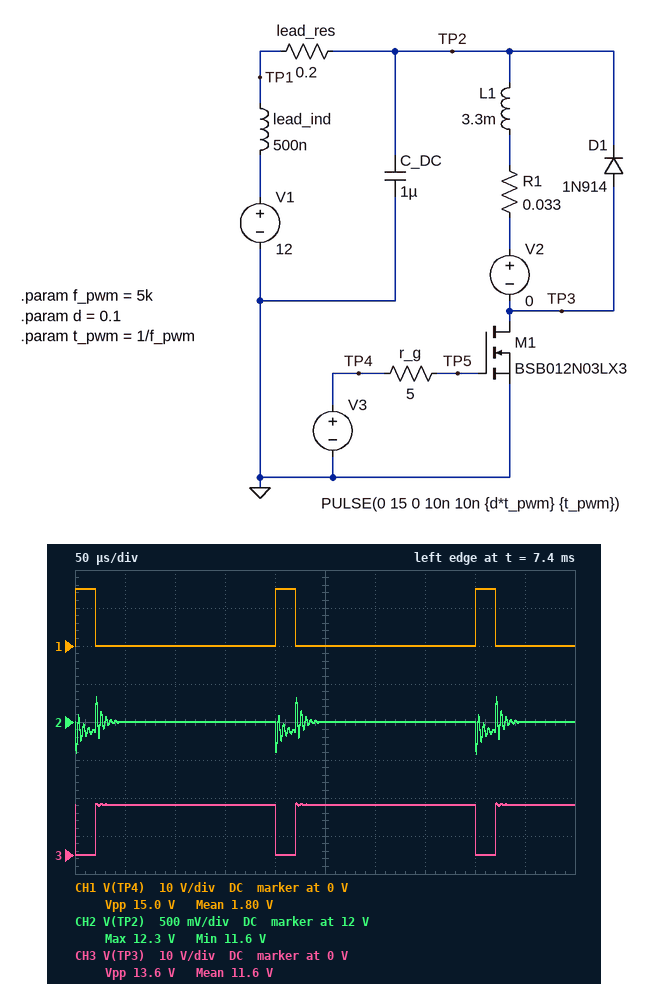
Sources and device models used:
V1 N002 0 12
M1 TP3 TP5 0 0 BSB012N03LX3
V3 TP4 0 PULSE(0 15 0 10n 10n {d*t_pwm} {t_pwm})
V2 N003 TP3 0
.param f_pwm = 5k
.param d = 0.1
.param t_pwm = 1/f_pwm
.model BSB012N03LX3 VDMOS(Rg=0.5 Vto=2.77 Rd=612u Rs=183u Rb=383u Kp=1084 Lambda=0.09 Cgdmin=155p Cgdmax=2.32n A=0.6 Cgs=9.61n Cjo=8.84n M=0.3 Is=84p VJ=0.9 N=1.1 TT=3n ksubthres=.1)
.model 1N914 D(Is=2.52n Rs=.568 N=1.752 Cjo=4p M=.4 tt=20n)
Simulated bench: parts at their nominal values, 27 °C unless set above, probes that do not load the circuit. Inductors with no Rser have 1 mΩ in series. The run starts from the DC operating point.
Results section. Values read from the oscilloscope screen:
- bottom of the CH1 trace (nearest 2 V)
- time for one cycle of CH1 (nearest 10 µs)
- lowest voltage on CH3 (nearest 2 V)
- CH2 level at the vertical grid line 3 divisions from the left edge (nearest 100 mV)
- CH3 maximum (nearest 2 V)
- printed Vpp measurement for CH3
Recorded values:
0 V
200 µs
0 V
12.0 V
14 V
13.6 V
